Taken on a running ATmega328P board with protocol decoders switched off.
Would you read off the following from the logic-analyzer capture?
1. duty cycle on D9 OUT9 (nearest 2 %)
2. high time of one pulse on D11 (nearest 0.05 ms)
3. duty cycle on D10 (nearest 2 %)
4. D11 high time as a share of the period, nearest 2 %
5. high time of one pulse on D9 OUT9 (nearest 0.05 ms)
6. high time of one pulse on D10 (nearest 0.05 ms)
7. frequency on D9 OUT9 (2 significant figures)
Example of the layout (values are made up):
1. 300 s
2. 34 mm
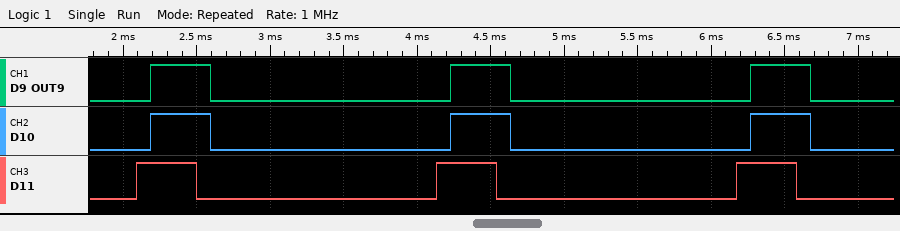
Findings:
1. 20 %
2. 0.40 ms
3. 20 %
4. 20 %
5. 0.40 ms
6. 0.40 ms
7. 490 Hz
